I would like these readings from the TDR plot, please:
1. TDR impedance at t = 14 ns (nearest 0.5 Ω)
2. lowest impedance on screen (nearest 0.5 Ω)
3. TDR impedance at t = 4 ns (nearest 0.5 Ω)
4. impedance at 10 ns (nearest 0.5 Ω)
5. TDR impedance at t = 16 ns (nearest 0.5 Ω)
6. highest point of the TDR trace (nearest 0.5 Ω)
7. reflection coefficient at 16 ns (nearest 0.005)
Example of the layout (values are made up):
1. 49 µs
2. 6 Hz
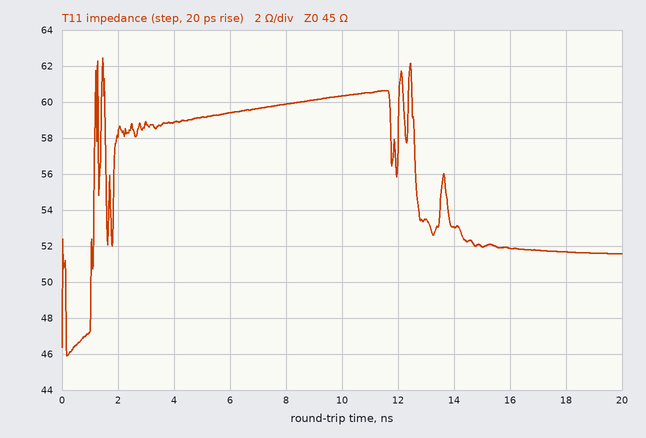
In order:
1. 53.0 Ω
2. 46.0 Ω
3. 59.0 Ω
4. 60.5 Ω
5. 52.0 Ω
6. 62.5 Ω
7. +0.070
